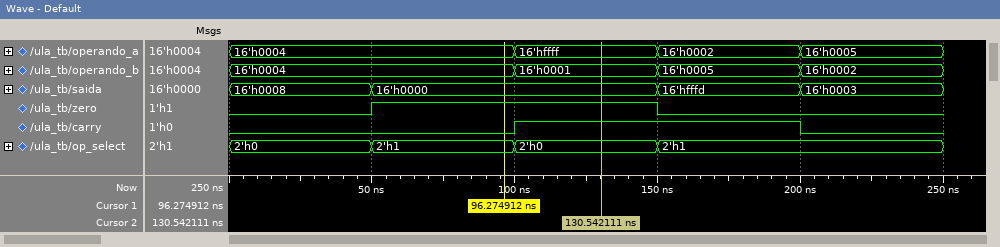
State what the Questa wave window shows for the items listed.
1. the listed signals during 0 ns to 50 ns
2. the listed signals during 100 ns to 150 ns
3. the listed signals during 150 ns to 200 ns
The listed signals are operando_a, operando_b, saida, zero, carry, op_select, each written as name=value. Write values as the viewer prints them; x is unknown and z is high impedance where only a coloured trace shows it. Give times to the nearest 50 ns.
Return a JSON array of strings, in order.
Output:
["operando_a=16'h0004, operando_b=16'h0004, saida=16'h0008, zero=0, carry=0, op_select=2'h0", "operando_a=16'hffff, operando_b=16'h0001, saida=16'h0000, zero=1, carry=1, op_select=2'h0", "operando_a=16'h0002, operando_b=16'h0005, saida=16'hfffd, zero=0, carry=1, op_select=2'h1"]
